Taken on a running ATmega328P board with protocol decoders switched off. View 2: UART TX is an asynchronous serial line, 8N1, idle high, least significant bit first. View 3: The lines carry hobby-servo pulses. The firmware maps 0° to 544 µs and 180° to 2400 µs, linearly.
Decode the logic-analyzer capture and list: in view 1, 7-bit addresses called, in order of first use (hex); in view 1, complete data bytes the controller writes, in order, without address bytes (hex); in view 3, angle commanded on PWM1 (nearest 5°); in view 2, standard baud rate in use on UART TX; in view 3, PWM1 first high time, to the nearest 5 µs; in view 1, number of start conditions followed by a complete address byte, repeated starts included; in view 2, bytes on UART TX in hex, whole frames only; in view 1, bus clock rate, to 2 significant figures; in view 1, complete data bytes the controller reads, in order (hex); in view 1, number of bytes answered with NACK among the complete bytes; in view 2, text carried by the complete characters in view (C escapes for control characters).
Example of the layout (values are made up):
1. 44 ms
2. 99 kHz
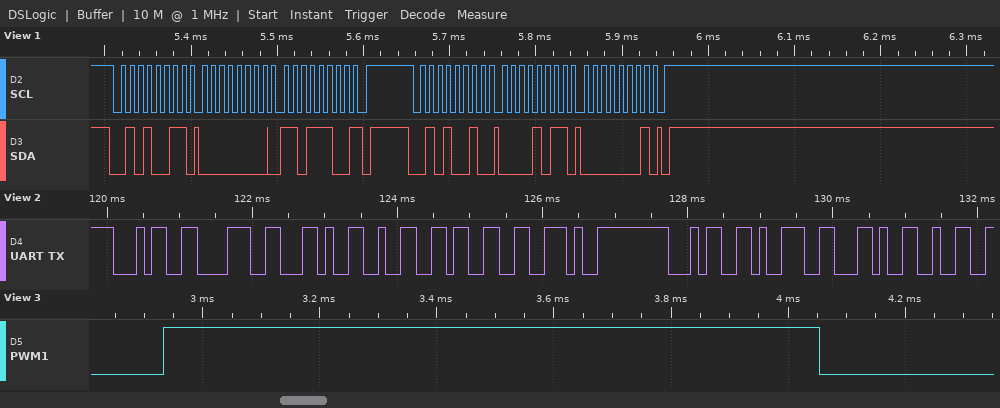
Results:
1. 0x29
2. 0B 01
3. 55°
4. 9600 baud
5. 1120 µs
6. 2
7. 0x34 0x38 0x2C 0x32 0x33 0x2E 0x34 0x39 0x2C 0x32
8. 100 kHz
9. 00 DC
10. 1
11. "48,23.49,2"
